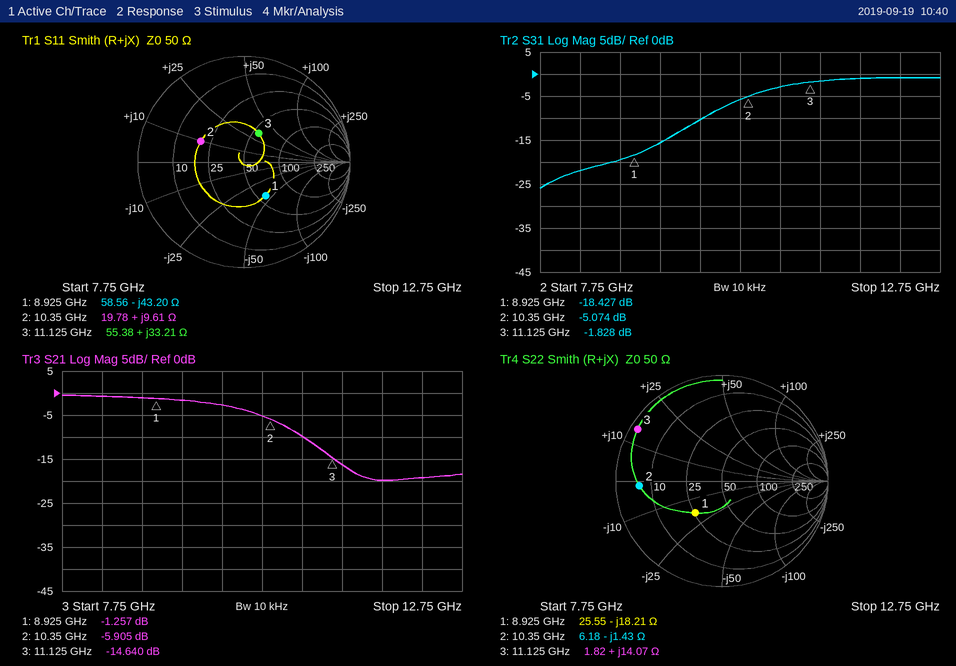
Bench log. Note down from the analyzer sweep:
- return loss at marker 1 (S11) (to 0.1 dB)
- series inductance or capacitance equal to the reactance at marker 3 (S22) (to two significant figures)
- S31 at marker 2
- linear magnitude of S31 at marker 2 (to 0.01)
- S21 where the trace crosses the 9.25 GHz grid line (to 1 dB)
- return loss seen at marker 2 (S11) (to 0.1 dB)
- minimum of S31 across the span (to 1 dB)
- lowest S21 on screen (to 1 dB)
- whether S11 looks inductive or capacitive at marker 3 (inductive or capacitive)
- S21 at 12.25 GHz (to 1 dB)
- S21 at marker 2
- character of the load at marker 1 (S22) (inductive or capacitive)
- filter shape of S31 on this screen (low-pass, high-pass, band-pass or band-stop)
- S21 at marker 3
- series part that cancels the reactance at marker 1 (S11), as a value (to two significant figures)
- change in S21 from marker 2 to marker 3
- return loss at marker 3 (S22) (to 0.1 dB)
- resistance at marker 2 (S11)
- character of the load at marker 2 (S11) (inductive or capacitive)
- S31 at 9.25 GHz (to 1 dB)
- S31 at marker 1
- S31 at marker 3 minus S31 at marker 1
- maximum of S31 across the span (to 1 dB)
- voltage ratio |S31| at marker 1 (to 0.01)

8.5 dB
200 pH
-5.074 dB
0.56
-2 dB
6.9 dB
-26 dB
-20 dB
inductive
-19 dB
-5.905 dB
capacitive
high-pass
-14.640 dB
770 pH
-8.735 dB
0.6 dB
19.78 Ω
inductive
-16 dB
-18.427 dB
16.599 dB
-1 dB
0.12
